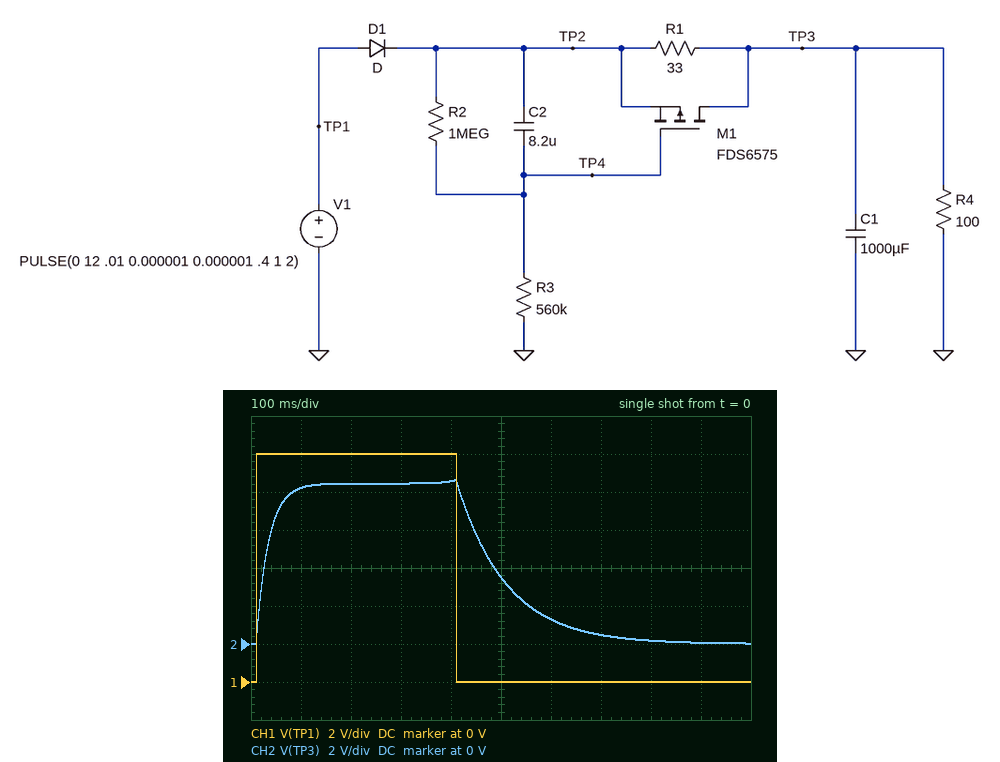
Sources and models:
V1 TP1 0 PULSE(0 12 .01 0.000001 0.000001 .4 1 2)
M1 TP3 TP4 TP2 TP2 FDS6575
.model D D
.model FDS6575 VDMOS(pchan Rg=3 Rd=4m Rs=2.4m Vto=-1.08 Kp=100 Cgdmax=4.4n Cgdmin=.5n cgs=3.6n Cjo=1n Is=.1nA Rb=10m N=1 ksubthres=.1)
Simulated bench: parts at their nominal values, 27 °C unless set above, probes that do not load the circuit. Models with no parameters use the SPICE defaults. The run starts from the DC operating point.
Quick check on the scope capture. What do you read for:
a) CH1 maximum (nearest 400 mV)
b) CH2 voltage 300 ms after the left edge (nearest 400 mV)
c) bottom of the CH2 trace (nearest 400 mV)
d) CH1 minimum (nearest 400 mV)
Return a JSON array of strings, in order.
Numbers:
["12.0 V", "8.4 V", "0 V", "0 V"]
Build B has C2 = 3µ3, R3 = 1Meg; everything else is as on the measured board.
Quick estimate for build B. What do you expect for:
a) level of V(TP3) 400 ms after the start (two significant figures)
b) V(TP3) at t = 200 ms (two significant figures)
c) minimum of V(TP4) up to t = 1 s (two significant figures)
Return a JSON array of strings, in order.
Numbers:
["11 V", "8.4 V", "-1.1 V"]
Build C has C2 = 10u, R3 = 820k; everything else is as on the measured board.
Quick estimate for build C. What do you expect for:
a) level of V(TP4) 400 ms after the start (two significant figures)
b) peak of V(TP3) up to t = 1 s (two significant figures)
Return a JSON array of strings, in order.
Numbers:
["11 V", "8.4 V"]
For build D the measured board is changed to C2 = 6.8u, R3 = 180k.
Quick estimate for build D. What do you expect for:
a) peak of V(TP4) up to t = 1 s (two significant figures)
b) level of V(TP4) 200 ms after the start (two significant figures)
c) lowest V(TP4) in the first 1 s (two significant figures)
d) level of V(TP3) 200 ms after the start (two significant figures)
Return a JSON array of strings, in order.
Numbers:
["11 V", "9.6 V", "-2.5 V", "11 V"]
